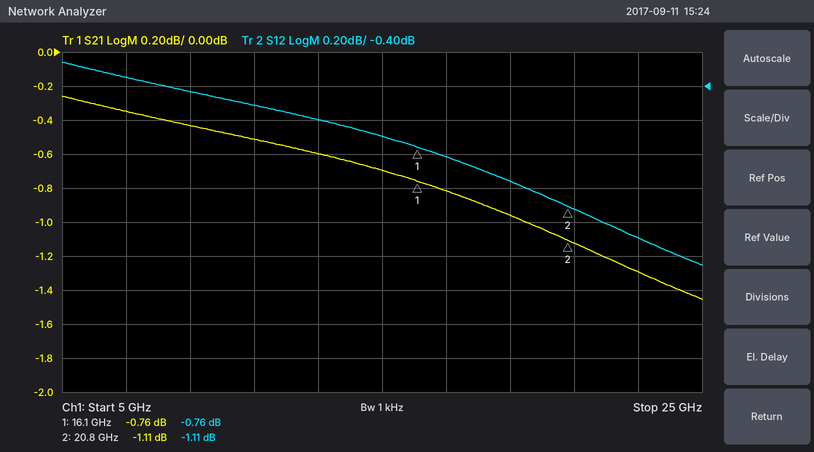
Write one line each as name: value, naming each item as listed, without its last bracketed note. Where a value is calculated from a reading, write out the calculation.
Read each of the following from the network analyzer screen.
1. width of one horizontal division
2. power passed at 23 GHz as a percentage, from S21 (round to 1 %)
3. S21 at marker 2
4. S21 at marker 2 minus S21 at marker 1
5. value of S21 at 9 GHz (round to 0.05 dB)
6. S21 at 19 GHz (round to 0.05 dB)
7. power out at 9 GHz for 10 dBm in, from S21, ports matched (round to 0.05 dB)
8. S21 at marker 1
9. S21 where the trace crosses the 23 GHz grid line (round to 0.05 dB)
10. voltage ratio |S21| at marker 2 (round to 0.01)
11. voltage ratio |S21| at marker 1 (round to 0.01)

width of one horizontal division: 2 GHz
power passed at 23 GHz as a percentage, from S21: 10^(-1.3/10) ≈ 74 %
S21 at marker 2: -1.11 dB
S21 at marker 2 minus S21 at marker 1: -1.11 − (-0.76) = -0.35 dB
value of S21 at 9 GHz: -0.45 dB
S21 at 19 GHz: -0.95 dB
power out at 9 GHz for 10 dBm in, from S21, ports matched: 10 dBm + (-0.45 dB) = 9.55 dBm
S21 at marker 1: -0.76 dB
S21 where the trace crosses the 23 GHz grid line: -1.30 dB
voltage ratio |S21| at marker 2: 10^(-1.11/20) ≈ 0.88
voltage ratio |S21| at marker 1: 10^(-0.76/20) ≈ 0.92
